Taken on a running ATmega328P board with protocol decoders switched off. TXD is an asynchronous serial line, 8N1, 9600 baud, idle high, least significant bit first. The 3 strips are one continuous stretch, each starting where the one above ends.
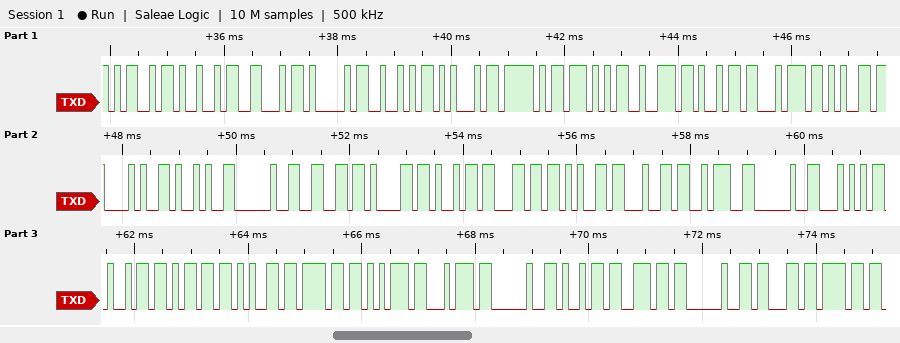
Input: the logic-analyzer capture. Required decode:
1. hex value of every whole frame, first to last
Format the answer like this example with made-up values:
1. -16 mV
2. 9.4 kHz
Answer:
1. 4D 49 46 41 52 45 5F 57 72 69 74 65 28 29 20 66 61 69 6C 65 64 3A 20 54 69 6D 65 6F 75 74 20 69 6E 20 63 6F
